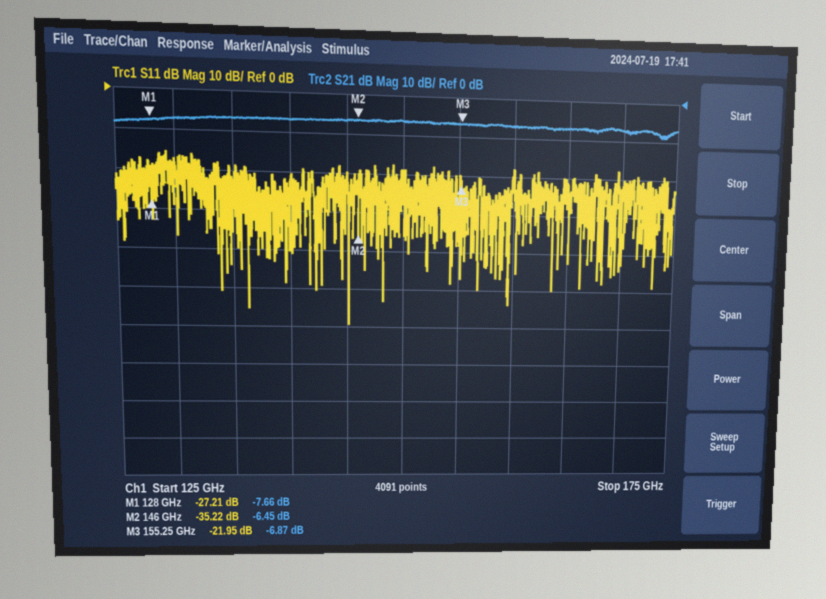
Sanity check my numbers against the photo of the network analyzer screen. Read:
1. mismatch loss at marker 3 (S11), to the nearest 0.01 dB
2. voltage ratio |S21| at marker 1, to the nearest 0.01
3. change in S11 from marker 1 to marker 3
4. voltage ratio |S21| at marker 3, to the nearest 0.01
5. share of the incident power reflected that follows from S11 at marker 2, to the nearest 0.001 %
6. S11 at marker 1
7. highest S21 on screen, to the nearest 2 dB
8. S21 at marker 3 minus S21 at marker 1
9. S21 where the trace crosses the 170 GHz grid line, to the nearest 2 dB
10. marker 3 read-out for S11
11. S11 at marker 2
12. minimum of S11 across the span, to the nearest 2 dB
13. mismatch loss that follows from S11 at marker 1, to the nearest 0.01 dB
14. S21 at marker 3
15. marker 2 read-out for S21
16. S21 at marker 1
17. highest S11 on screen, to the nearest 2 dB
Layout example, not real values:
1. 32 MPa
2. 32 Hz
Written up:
1. 0.03 dB
2. 0.41
3. 5.26 dB
4. 0.45
5. 0.030 %
6. -27.21 dB
7. -6 dB
8. 0.79 dB
9. -8 dB
10. -21.95 dB
11. -35.22 dB
12. -60 dB
13. 0.01 dB
14. -6.87 dB
15. -6.45 dB
16. -7.66 dB
17. -16 dB
